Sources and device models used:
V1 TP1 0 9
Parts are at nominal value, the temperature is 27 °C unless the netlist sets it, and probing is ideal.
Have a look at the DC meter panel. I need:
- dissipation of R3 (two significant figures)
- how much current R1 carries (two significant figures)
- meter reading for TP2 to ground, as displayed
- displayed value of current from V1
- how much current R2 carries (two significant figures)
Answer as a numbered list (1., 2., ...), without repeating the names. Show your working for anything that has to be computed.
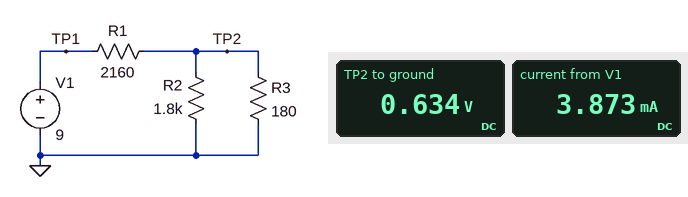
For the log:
1. (634 mV)^2 / 180 Ω = 2.2 mW
2. (9 V - 634 mV) / 2.16 kΩ = 3.9 mA
3. 0.634 V
4. 3.873 mA
5. (634 mV) / 1.8 kΩ = 350 µA
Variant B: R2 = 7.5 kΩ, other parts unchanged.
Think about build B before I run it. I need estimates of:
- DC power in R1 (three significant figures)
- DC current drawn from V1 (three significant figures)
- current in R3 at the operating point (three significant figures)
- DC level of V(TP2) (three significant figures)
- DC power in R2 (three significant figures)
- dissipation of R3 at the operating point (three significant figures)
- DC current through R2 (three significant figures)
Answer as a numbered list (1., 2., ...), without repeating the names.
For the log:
1. 32.1 mW
2. 3.85 mA
3. 3.76 mA
4. 677 mV
5. 61.2 µW
6. 2.55 mW
7. 90.3 µA
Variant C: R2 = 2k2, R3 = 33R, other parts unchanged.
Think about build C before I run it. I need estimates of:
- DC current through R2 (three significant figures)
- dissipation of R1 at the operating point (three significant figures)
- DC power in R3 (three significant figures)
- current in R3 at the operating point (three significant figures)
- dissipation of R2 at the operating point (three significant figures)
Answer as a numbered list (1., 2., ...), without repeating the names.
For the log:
1. 60.7 µA
2. 36.4 mW
3. 540 µW
4. 4.04 mA
5. 8.10 µW
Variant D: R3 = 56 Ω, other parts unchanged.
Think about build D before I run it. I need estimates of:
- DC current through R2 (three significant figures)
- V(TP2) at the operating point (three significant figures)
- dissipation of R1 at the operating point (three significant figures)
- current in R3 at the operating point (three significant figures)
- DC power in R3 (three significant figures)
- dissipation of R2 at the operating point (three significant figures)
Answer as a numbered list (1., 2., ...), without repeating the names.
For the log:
1. 123 µA
2. 221 mV
3. 35.7 mW
4. 3.94 mA
5. 870 µW
6. 27.1 µW
